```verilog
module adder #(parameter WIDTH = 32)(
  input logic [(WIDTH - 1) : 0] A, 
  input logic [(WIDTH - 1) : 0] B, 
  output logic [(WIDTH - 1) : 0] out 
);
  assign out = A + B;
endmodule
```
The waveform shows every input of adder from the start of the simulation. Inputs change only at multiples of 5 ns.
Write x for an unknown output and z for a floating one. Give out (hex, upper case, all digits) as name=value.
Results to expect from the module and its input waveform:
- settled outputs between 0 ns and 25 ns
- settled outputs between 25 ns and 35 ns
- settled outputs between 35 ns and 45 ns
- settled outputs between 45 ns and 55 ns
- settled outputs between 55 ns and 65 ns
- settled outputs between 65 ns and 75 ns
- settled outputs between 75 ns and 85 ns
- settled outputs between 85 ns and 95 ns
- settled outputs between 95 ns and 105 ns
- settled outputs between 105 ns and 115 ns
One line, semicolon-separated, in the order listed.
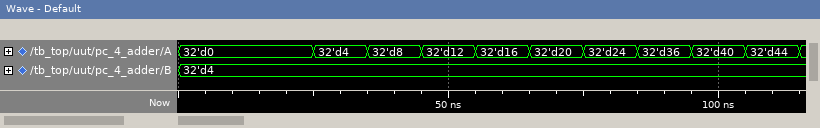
out=00000004; out=00000008; out=0000000C; out=00000010; out=00000014; out=00000018; out=0000001C; out=00000028; out=0000002C; out=00000030
